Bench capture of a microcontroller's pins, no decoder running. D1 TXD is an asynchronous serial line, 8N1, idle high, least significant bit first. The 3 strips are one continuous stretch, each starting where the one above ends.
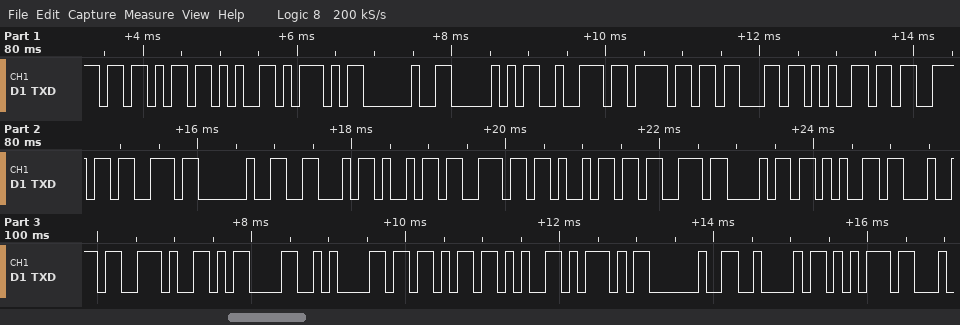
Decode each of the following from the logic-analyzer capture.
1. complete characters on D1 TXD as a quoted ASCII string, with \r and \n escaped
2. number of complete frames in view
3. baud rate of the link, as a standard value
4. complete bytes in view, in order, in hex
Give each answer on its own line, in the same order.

"[+] Process Finished.\r\n[+] Bu"
29
9600 baud
5B 2B 5D 20 50 72 6F 63 65 73 73 20 46 69 6E 69 73 68 65 64 2E 0D 0A 5B 2B 5D 20 42 75
